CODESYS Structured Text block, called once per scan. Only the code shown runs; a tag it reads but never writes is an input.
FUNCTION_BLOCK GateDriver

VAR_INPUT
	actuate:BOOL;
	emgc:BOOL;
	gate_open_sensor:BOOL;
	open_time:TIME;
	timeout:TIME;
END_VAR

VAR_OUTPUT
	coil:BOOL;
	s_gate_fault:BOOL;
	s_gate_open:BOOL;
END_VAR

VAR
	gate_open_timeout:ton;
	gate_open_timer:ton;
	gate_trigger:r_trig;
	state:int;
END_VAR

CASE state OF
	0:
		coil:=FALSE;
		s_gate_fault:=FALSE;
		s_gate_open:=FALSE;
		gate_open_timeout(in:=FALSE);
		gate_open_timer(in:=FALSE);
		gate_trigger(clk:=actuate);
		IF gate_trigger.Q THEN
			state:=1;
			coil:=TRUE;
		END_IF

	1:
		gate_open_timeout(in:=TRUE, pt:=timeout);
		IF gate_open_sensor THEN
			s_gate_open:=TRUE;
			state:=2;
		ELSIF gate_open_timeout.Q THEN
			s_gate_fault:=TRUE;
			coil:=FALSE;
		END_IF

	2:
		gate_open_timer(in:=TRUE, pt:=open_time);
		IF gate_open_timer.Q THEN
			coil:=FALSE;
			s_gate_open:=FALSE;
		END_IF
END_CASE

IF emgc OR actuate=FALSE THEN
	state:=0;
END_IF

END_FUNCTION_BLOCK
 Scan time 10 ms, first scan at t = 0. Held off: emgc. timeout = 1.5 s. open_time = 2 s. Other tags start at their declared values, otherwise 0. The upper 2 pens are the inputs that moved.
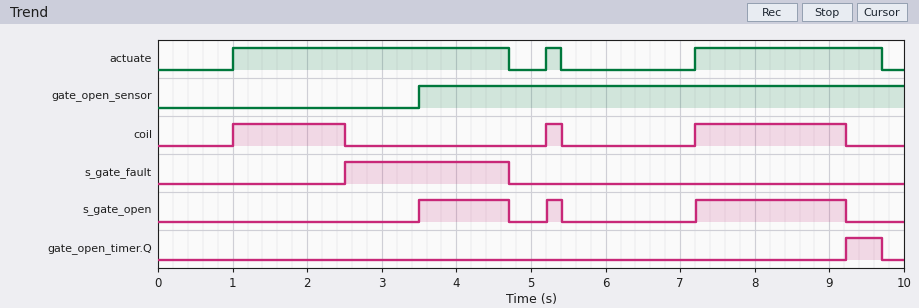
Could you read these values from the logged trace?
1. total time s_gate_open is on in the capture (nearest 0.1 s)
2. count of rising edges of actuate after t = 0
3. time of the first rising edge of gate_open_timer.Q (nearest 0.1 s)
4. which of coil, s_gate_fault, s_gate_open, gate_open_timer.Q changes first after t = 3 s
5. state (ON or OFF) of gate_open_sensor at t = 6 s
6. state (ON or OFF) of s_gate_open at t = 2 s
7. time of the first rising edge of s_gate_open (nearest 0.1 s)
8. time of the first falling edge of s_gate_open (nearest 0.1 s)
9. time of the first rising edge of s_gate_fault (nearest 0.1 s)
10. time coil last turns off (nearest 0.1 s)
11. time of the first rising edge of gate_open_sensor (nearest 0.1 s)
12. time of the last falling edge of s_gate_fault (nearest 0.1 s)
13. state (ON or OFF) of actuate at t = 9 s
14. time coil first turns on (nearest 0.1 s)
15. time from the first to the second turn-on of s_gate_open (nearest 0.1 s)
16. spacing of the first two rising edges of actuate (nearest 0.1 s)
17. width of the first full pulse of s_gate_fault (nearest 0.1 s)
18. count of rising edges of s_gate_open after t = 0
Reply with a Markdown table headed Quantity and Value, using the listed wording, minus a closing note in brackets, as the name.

| Quantity | Value |
|---|---|
| total time s_gate_open is on in the capture | 3.4 s |
| count of rising edges of actuate after t = 0 | 3 |
| time of the first rising edge of gate_open_timer.Q | 9.2 s |
| which of coil, s_gate_fault, s_gate_open, gate_open_timer.Q changes first after t = 3 s | s_gate_open |
| state (ON or OFF) of gate_open_sensor at t = 6 s | ON |
| state (ON or OFF) of s_gate_open at t = 2 s | OFF |
| time of the first rising edge of s_gate_open | 3.5 s |
| time of the first falling edge of s_gate_open | 4.7 s |
| time of the first rising edge of s_gate_fault | 2.5 s |
| time coil last turns off | 9.2 s |
| time of the first rising edge of gate_open_sensor | 3.5 s |
| time of the last falling edge of s_gate_fault | 4.7 s |
| state (ON or OFF) of actuate at t = 9 s | ON |
| time coil first turns on | 1.0 s |
| time from the first to the second turn-on of s_gate_open | 1.7 s |
| spacing of the first two rising edges of actuate | 4.2 s |
| width of the first full pulse of s_gate_fault | 2.2 s |
| count of rising edges of s_gate_open after t = 0 | 3 |
